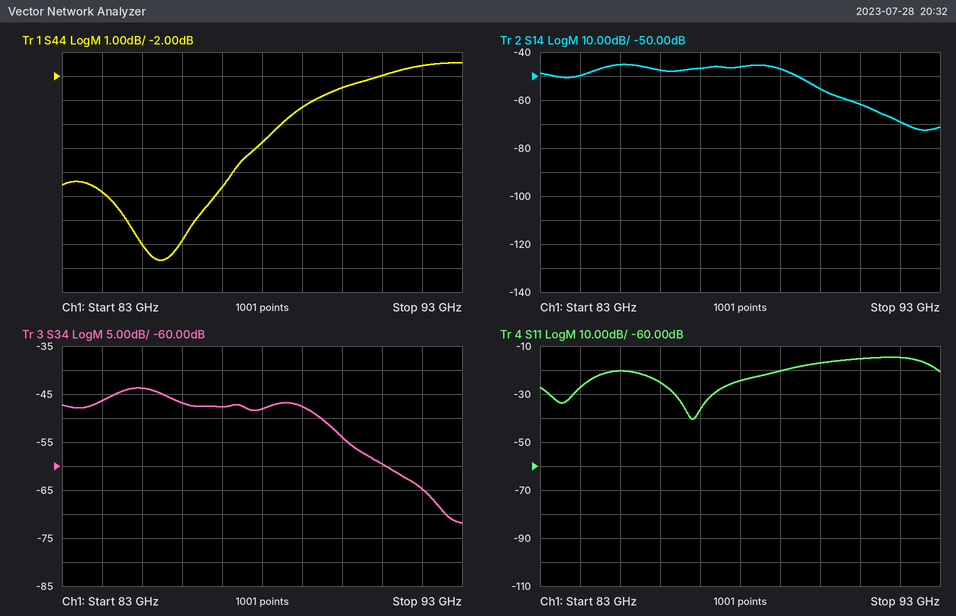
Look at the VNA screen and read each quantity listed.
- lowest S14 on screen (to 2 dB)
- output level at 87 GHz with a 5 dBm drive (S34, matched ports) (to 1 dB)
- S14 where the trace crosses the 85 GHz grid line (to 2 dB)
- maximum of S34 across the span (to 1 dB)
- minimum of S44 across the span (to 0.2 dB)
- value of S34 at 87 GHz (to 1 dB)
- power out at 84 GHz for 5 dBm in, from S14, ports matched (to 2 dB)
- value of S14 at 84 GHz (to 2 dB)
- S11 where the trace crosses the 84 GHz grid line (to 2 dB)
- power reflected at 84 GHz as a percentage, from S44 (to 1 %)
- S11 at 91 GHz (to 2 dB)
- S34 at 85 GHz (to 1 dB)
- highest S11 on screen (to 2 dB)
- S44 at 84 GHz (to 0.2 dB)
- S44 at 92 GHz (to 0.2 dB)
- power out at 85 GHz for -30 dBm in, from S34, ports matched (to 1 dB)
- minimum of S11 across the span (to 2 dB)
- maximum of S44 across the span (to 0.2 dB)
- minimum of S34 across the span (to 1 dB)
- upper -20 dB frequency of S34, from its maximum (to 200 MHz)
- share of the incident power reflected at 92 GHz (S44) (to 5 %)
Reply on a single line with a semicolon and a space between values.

-72 dB; -43 dBm; -46 dB; -44 dB; -9.6 dB; -48 dB; -44 dBm; -50 dB; -28 dB; 21 %; -16 dB; -44 dB; -14 dB; -6.8 dB; -1.6 dB; -74 dBm; -40 dB; -1.4 dB; -72 dB; 91.8 GHz; 70 %
